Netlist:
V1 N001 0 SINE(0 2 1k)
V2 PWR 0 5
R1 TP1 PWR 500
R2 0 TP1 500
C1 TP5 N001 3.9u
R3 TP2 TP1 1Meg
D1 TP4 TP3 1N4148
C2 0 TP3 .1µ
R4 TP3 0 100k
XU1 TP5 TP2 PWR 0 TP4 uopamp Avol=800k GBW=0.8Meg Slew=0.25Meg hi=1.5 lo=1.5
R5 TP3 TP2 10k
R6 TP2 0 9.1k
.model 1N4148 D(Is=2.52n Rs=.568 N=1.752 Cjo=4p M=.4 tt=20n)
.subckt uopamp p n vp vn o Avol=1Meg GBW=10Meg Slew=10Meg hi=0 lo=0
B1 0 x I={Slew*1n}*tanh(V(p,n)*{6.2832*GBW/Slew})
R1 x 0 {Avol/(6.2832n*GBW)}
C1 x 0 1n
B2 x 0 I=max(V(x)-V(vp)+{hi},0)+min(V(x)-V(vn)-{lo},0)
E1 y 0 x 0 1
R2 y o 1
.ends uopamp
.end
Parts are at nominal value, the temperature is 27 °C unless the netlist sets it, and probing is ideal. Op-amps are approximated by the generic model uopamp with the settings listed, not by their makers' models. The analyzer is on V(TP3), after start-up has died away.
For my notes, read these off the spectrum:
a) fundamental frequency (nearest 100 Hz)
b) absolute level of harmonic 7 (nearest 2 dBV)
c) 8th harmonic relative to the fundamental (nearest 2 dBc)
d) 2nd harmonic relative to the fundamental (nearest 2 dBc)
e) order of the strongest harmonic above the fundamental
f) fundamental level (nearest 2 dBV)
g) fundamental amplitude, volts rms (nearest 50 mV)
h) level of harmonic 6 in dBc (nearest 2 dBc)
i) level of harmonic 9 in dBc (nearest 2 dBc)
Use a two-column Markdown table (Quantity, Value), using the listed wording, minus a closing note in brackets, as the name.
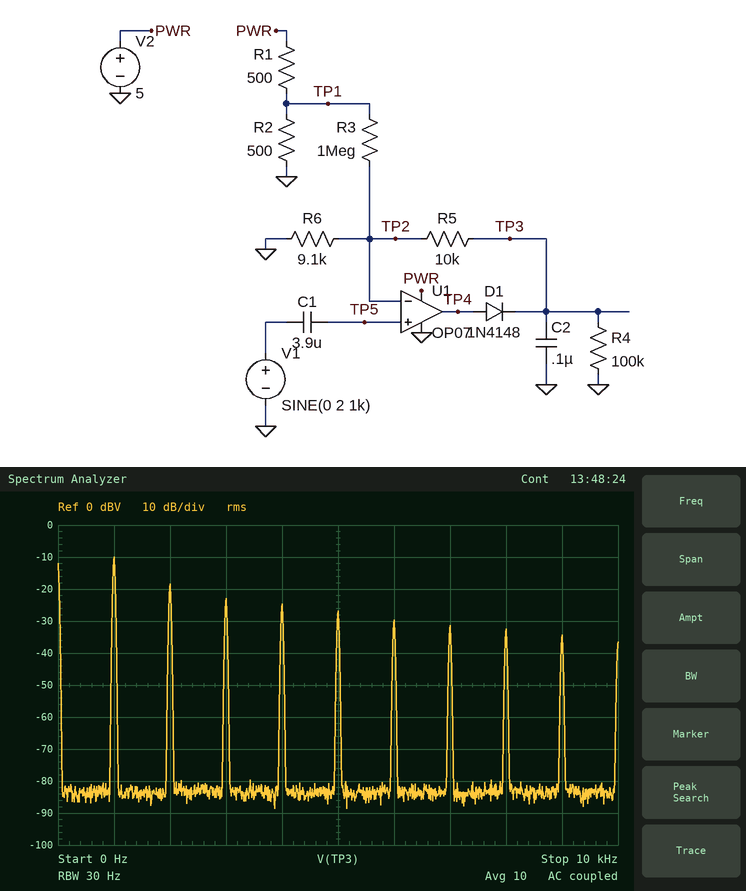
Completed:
| Quantity | Value |
|---|---|
| fundamental frequency | 1.0 kHz |
| absolute level of harmonic 7 | -32 dBV |
| 8th harmonic relative to the fundamental | -22 dBc |
| 2nd harmonic relative to the fundamental | -8 dBc |
| order of the strongest harmonic above the fundamental | 2 |
| fundamental level | -10 dBV |
| fundamental amplitude, volts rms | 300 mV |
| level of harmonic 6 in dBc | -20 dBc |
| level of harmonic 9 in dBc | -24 dBc |
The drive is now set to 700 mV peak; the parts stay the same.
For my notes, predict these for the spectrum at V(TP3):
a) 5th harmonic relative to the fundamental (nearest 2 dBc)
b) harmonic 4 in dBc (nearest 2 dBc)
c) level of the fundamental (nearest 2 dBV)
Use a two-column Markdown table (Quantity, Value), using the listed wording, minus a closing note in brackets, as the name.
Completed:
| Quantity | Value |
|---|---|
| 5th harmonic relative to the fundamental | -20 dBc |
| harmonic 4 in dBc | -16 dBc |
| level of the fundamental | -18 dBV |
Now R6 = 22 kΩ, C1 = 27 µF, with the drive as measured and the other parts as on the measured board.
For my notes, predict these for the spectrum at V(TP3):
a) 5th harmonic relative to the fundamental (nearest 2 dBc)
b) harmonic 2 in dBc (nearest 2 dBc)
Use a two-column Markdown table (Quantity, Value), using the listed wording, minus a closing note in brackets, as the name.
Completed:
| Quantity | Value |
|---|---|
| 5th harmonic relative to the fundamental | -18 dBc |
| harmonic 2 in dBc | -6 dBc |
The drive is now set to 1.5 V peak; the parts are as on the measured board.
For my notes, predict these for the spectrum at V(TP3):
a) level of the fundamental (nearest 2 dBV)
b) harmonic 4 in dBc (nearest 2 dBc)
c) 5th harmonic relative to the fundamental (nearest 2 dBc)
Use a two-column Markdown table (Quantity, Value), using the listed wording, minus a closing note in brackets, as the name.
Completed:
| Quantity | Value |
|---|---|
| level of the fundamental | -10 dBV |
| harmonic 4 in dBc | -16 dBc |
| 5th harmonic relative to the fundamental | -20 dBc |
